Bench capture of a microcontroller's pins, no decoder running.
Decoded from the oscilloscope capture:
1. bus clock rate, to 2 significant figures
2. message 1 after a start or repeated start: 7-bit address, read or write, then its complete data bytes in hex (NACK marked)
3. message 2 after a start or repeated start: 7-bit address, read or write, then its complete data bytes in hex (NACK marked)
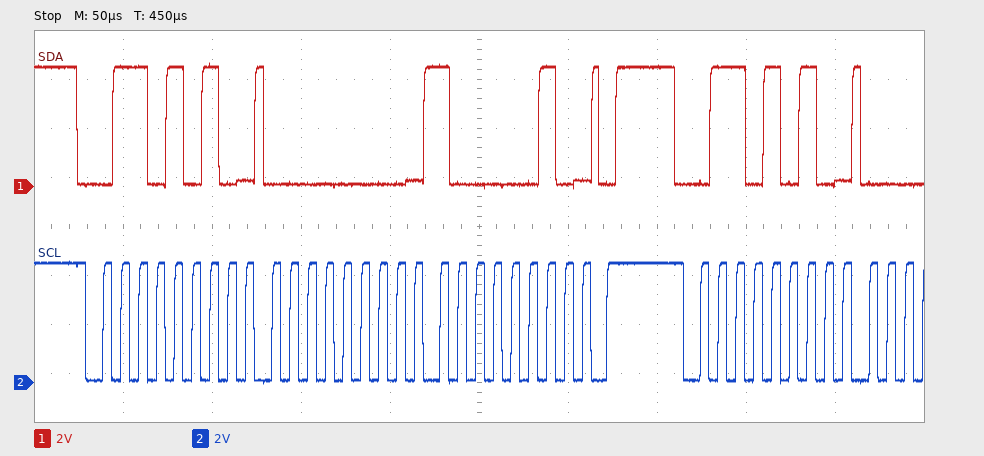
100 kHz
0x35 write: 00 82
0x35 write
